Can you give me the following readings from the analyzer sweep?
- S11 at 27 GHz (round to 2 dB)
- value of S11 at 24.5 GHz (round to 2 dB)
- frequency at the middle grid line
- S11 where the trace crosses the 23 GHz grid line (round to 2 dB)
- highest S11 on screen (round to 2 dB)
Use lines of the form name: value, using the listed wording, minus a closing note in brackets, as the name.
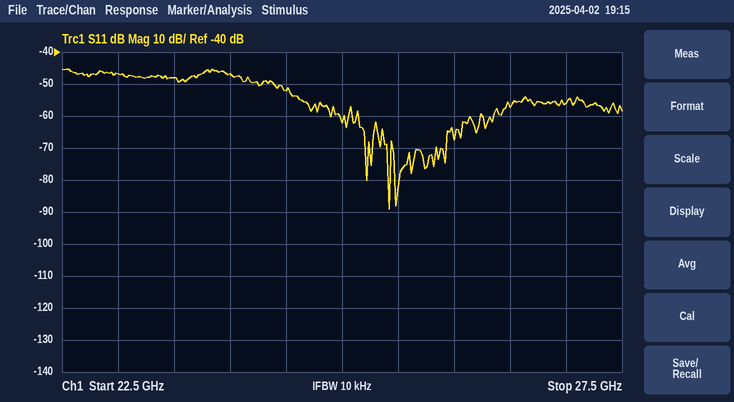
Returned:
S11 at 27 GHz: -56 dB
value of S11 at 24.5 GHz: -52 dB
frequency at the middle grid line: 25 GHz
S11 where the trace crosses the 23 GHz grid line: -46 dB
highest S11 on screen: -46 dB
